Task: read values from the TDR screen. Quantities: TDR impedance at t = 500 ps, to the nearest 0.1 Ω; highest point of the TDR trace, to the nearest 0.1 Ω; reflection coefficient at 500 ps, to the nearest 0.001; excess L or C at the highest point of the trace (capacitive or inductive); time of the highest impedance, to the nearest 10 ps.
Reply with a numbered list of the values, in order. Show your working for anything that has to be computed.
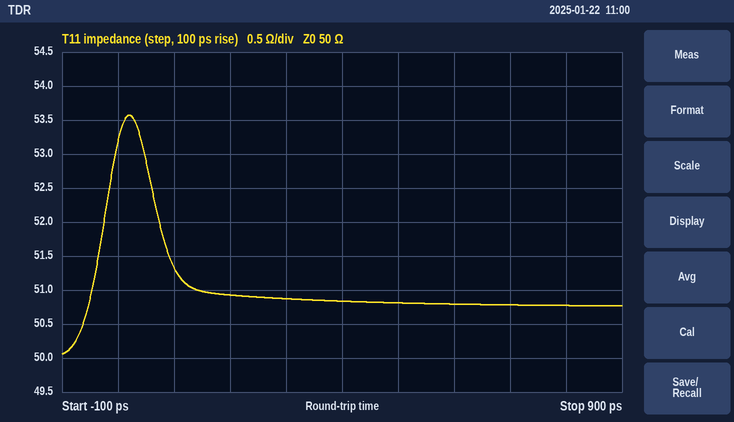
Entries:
1. 50.8 Ω
2. 53.6 Ω
3. (50.8 − 50)/(50.8 + 50) ≈ +0.008
4. inductive
5. 20 ps
